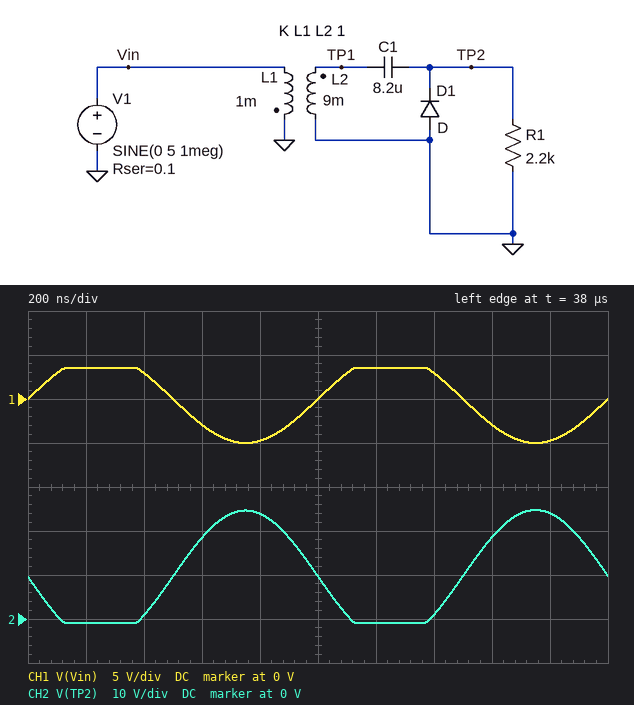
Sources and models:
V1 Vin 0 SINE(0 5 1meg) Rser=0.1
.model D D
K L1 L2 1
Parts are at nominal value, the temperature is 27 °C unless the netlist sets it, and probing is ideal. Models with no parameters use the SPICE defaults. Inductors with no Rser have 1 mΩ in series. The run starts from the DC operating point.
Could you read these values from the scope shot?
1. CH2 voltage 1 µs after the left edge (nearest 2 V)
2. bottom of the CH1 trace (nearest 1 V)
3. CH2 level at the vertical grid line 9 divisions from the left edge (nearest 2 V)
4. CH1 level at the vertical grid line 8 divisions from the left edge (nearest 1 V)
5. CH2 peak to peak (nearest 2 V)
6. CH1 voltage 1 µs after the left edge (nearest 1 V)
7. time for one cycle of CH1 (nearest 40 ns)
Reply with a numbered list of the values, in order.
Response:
1. 10 V
2. -5 V
3. 24 V
4. -3 V
5. 26 V
6. 0 V
7. 1.00 µs
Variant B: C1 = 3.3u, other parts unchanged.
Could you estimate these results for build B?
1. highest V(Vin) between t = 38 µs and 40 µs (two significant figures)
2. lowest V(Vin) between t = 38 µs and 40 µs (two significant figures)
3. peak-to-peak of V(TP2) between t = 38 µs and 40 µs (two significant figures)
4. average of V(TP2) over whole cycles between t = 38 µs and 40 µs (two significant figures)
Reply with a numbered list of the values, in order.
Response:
1. 4.5 V
2. -5.0 V
3. 28 V
4. 13 V
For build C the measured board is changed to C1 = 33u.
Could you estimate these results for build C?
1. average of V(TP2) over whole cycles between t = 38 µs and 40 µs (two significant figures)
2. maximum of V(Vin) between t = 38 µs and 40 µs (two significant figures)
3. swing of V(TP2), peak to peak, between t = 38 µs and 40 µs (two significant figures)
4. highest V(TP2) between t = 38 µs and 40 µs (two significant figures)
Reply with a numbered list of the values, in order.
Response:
1. 6.8 V
2. 1.8 V
3. 20 V
4. 19 V
